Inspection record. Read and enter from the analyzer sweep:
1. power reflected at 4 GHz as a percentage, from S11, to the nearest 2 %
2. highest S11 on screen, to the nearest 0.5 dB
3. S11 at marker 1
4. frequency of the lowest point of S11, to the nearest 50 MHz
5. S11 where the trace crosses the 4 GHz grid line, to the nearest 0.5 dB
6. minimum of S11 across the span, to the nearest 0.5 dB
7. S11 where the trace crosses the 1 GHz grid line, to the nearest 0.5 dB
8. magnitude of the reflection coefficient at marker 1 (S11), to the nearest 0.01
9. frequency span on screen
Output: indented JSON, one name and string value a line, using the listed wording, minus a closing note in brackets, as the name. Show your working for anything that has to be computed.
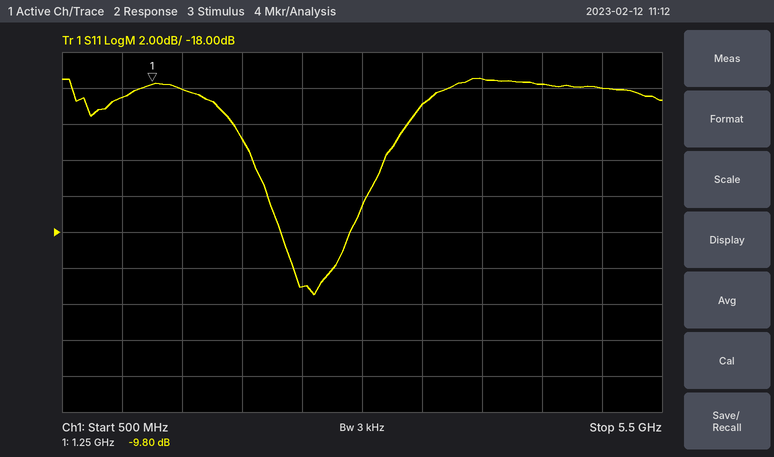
{
  "power reflected at 4 GHz as a percentage, from S11, to the nearest 2 %": "10^(-9.5/10) ≈ 11.2 %, so 12 % to the nearest 2 %",
  "highest S11 on screen, to the nearest 0.5 dB": "-9.5 dB",
  "S11 at marker 1": "-9.80 dB",
  "frequency of the lowest point of S11, to the nearest 50 MHz": "2.60 GHz",
  "S11 where the trace crosses the 4 GHz grid line, to the nearest 0.5 dB": "-9.5 dB",
  "minimum of S11 across the span, to the nearest 0.5 dB": "-21.5 dB",
  "S11 where the trace crosses the 1 GHz grid line, to the nearest 0.5 dB": "-10.5 dB",
  "magnitude of the reflection coefficient at marker 1 (S11), to the nearest 0.01": "10^(-9.8/20) ≈ 0.32",
  "frequency span on screen": "5 GHz"
}
